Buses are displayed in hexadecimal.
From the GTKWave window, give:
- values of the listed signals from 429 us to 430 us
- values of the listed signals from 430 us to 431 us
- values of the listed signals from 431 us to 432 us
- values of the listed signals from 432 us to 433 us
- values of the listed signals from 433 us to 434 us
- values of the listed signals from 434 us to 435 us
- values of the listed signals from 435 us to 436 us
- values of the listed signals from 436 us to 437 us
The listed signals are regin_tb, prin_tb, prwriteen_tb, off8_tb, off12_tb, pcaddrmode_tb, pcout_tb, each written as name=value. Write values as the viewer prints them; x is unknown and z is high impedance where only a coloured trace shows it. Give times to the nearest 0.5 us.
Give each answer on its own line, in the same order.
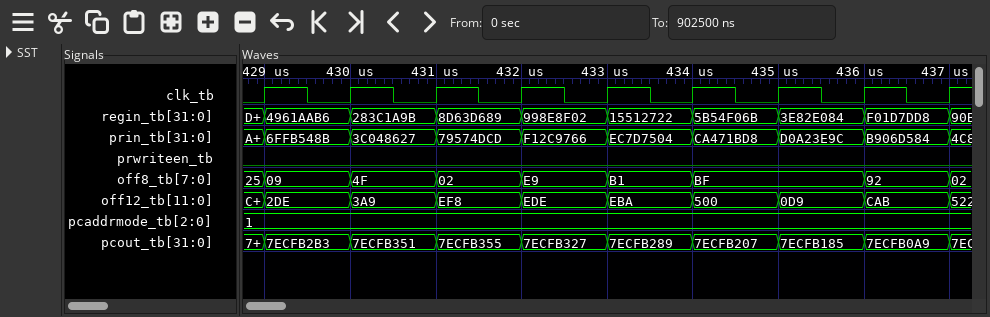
regin_tb=4961AAB6, prin_tb=6FFB548B, prwriteen_tb=0, off8_tb=09, off12_tb=2DE, pcaddrmode_tb=1, pcout_tb=7ECFB2B3
regin_tb=283C1A9B, prin_tb=3C048627, prwriteen_tb=0, off8_tb=4F, off12_tb=3A9, pcaddrmode_tb=1, pcout_tb=7ECFB351
regin_tb=8D63D689, prin_tb=79574DCD, prwriteen_tb=0, off8_tb=02, off12_tb=EF8, pcaddrmode_tb=1, pcout_tb=7ECFB355
regin_tb=998E8F02, prin_tb=F12C9766, prwriteen_tb=0, off8_tb=E9, off12_tb=EDE, pcaddrmode_tb=1, pcout_tb=7ECFB327
regin_tb=15512722, prin_tb=EC7D7504, prwriteen_tb=0, off8_tb=B1, off12_tb=EBA, pcaddrmode_tb=1, pcout_tb=7ECFB289
regin_tb=5B54F06B, prin_tb=CA471BD8, prwriteen_tb=0, off8_tb=BF, off12_tb=500, pcaddrmode_tb=1, pcout_tb=7ECFB207
regin_tb=3E82E084, prin_tb=D0A23E9C, prwriteen_tb=0, off8_tb=BF, off12_tb=0D9, pcaddrmode_tb=1, pcout_tb=7ECFB185
regin_tb=F01D7DD8, prin_tb=B906D584, prwriteen_tb=0, off8_tb=92, off12_tb=CAB, pcaddrmode_tb=1, pcout_tb=7ECFB0A9
